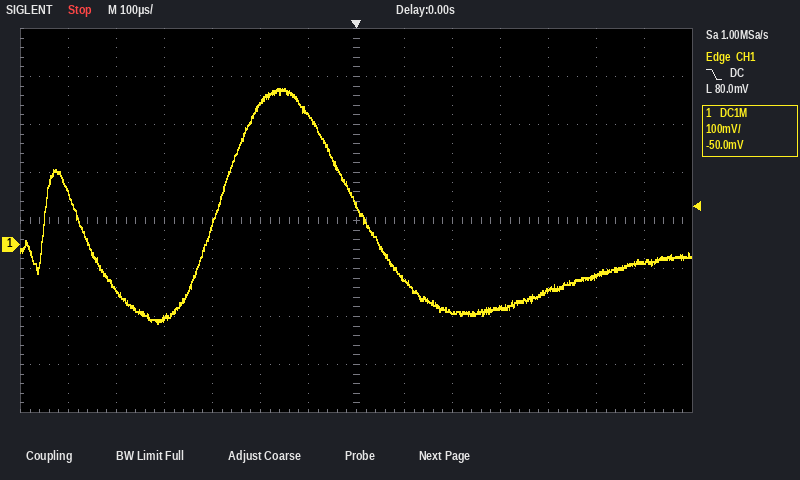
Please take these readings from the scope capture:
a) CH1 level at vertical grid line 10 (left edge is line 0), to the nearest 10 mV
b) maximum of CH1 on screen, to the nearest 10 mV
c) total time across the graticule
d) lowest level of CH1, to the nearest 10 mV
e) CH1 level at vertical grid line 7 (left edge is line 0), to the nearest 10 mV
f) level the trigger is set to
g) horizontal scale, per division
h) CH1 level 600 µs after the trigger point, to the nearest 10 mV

-130 mV
320 mV
1.4 ms
-160 mV
80 mV
80.0 mV
100 µs
-40 mV
